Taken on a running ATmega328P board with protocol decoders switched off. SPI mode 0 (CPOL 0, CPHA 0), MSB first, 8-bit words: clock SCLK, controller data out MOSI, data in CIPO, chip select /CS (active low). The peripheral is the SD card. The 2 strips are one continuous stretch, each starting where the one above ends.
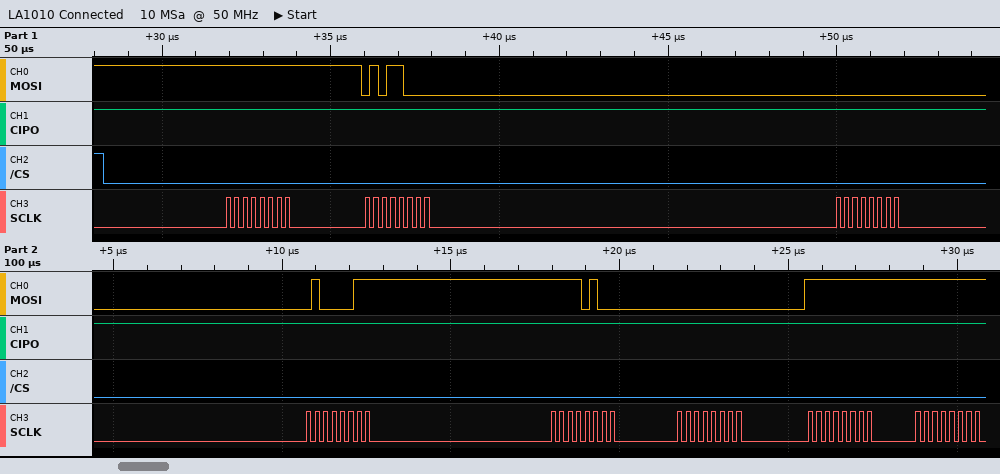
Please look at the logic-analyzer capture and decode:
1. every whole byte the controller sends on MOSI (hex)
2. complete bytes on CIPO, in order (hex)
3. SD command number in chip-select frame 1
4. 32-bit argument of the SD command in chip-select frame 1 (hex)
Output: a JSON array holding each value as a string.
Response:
["0xFF 0x58 0x00 0x43 0xF4 0x00 0xFF 0xFF", "0xFF 0xFF 0xFF 0xFF 0xFF 0xFF 0xFF 0xFF", "CMD24", "0x0043F400"]
